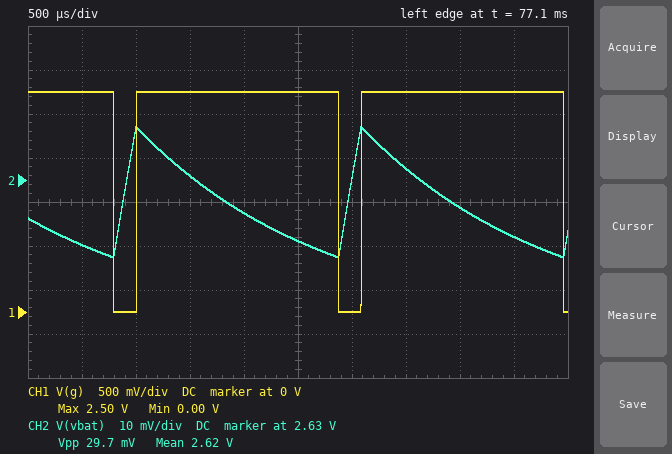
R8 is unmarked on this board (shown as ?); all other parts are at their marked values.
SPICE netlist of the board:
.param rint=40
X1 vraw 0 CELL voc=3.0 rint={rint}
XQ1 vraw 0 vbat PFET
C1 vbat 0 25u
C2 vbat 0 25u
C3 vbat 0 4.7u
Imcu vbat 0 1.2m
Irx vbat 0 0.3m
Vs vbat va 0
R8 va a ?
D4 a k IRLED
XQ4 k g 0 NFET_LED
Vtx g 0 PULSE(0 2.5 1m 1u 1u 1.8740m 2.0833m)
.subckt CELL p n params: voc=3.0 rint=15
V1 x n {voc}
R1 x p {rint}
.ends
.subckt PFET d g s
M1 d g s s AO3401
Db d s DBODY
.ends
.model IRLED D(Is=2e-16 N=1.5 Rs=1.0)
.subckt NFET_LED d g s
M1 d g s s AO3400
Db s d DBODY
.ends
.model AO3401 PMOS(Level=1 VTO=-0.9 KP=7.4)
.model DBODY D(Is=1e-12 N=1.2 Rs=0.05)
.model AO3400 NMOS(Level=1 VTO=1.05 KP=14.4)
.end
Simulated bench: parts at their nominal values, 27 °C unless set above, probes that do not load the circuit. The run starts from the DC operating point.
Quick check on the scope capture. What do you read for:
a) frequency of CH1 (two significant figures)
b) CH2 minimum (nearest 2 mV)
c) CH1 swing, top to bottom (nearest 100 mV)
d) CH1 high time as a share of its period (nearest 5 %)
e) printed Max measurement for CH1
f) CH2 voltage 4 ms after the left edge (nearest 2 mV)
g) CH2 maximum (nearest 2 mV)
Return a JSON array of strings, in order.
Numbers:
["480 Hz", "2.612 V", "2.5 V", "90 %", "2.50 V", "2.624 V", "2.642 V"]
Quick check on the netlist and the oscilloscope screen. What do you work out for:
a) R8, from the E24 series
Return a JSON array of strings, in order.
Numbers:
["160 Ω"]
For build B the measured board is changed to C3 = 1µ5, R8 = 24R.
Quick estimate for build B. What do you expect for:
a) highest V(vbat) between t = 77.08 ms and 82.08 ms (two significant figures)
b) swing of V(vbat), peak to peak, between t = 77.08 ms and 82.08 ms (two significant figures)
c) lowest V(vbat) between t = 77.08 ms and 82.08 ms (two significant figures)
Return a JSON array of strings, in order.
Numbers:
["2.0 V", "98 mV", "1.9 V"]
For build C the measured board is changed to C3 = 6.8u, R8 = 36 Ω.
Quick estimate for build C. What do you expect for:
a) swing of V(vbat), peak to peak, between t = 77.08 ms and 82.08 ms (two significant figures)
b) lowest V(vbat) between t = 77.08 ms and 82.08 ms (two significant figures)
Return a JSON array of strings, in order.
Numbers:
["75 mV", "2.1 V"]
